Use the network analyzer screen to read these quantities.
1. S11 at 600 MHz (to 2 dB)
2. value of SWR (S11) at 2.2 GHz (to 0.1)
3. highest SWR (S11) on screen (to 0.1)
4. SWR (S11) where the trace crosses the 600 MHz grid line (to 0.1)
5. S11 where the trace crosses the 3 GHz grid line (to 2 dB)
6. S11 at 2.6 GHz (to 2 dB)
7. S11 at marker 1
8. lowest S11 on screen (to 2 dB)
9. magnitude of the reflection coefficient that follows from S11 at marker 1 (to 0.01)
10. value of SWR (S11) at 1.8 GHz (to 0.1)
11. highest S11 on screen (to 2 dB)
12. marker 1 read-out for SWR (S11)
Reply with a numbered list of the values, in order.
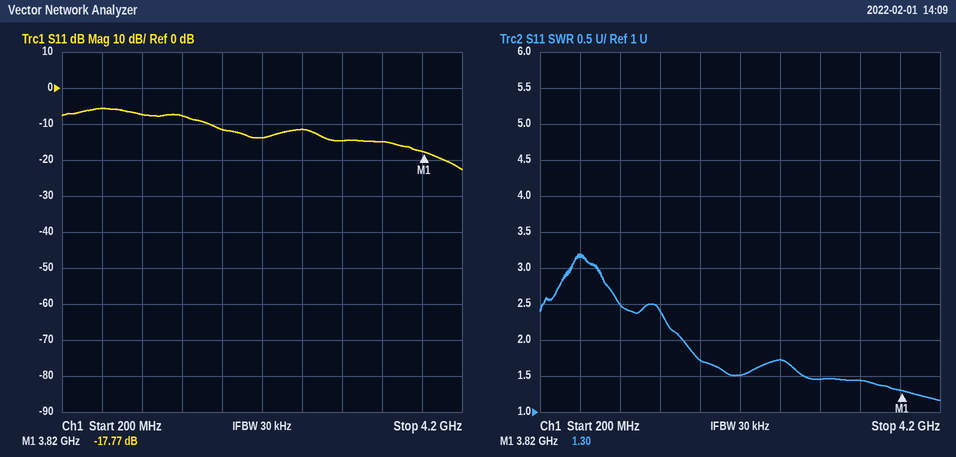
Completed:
1. -6 dB
2. 1.5
3. 3.2
4. 3.2
5. -14 dB
6. -12 dB
7. -17.77 dB
8. -22 dB
9. 0.13
10. 1.7
11. -6 dB
12. 1.30
